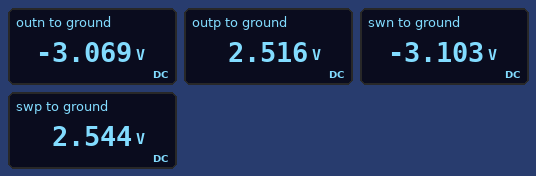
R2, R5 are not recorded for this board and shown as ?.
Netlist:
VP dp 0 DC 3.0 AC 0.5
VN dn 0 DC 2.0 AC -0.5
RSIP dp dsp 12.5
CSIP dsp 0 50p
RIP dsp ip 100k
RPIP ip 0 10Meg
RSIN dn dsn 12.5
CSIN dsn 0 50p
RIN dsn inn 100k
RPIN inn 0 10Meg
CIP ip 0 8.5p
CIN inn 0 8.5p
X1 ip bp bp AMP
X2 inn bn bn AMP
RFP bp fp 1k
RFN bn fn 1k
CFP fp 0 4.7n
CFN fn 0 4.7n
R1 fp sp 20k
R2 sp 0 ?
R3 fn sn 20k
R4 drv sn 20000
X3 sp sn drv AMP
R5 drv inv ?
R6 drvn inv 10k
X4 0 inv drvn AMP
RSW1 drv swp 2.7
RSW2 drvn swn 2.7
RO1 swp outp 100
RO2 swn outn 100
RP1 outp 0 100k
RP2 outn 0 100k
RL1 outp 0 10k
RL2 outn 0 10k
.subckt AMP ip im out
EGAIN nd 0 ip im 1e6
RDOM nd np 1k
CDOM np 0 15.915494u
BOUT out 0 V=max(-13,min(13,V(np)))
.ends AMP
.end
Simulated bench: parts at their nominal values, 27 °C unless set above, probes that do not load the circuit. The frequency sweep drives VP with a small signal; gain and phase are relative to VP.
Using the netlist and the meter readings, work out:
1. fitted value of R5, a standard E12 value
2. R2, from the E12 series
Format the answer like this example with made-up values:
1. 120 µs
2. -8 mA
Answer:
1. 8.2 kΩ
2. 68 kΩ
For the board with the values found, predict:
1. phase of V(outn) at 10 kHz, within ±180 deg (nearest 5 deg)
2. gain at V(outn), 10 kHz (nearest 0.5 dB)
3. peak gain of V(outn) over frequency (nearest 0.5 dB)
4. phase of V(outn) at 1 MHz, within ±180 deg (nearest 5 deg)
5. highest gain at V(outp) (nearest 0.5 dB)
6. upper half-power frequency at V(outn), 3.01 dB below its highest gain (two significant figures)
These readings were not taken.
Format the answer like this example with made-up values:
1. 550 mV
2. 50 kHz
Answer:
1. 160 deg
2. 7.0 dB
3. 7.5 dB
4. -15 deg
5. 5.5 dB
6. 34 kHz
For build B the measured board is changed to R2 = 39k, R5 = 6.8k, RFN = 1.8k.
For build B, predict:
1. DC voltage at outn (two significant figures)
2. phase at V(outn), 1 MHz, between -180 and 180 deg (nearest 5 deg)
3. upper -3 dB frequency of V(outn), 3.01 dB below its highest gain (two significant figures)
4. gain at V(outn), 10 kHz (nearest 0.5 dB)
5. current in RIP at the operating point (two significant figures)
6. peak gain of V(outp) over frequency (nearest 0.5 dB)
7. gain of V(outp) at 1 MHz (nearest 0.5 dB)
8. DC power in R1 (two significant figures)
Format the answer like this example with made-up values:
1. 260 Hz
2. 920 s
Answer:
1. -2.7 V
2. -20 deg
3. 30 kHz
4. 7.5 dB
5. 300 nA
6. 4.5 dB
7. -40.5 dB
8. 49 µW
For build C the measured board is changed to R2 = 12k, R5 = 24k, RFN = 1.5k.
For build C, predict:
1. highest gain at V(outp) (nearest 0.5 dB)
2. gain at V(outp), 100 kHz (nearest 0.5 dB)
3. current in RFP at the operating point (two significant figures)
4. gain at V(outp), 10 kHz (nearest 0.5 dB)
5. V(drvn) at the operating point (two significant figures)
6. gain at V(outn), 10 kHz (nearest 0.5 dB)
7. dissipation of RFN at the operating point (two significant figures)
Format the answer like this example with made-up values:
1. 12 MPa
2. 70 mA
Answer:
1. 1.0 dB
2. -10.5 dB
3. 90 µA
4. 0.5 dB
5. -100 mV
6. -7.0 dB
7. 2.6 µW
